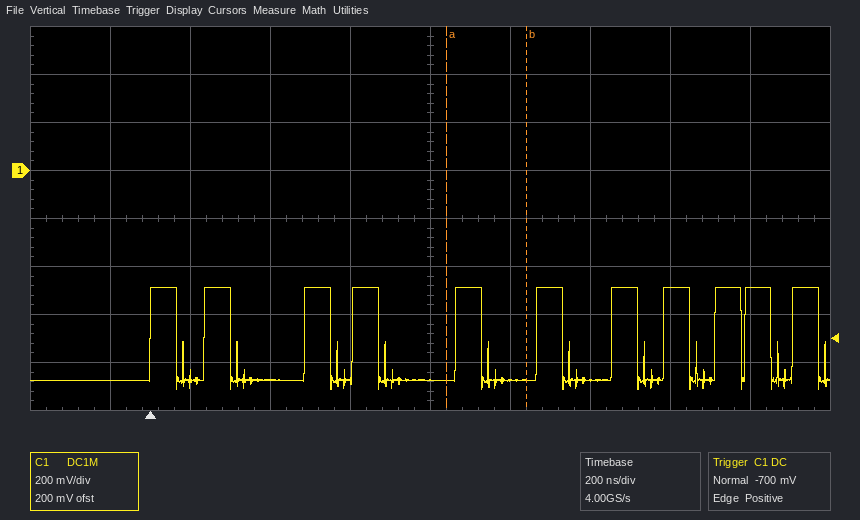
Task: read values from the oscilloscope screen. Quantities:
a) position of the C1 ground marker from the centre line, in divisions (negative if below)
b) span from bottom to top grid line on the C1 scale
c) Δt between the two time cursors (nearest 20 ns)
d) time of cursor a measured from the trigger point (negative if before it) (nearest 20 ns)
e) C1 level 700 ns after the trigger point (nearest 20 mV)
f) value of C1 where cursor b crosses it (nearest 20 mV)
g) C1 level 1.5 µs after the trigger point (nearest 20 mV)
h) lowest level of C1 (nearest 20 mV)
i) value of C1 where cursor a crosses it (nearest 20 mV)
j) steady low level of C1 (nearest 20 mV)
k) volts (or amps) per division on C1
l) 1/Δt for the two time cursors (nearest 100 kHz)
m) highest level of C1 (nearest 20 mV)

+1.0 div
1.6 V
200 ns
+740 ns
-880 mV
-880 mV
-480 mV
-920 mV
-880 mV
-880 mV
200 mV
5.0 MHz
-480 mV
